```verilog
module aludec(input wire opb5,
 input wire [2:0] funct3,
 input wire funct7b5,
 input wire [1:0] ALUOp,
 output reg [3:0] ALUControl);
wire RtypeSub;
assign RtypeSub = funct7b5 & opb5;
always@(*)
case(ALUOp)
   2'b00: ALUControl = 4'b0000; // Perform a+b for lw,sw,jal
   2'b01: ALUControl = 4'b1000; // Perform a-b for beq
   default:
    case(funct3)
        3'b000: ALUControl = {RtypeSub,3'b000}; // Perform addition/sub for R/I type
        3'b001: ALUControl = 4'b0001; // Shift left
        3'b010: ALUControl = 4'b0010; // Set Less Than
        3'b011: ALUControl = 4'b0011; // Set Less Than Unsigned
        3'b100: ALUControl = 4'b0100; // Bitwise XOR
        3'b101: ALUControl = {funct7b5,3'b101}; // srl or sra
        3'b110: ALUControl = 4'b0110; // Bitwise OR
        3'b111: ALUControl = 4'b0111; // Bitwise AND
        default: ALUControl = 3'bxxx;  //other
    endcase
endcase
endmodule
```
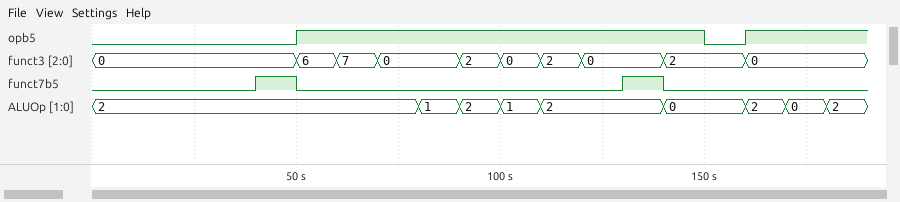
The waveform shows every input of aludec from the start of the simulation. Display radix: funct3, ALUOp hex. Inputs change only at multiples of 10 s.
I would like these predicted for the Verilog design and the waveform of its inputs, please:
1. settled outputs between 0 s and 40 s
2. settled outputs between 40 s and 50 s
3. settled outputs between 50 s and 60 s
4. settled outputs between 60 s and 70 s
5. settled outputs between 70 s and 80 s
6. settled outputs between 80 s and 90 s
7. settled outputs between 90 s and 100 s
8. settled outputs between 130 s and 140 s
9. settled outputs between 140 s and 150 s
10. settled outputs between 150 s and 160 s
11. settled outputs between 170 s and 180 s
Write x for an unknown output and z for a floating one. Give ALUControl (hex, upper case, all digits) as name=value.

ALUControl=0
ALUControl=0
ALUControl=6
ALUControl=7
ALUControl=0
ALUControl=8
ALUControl=2
ALUControl=8
ALUControl=0
ALUControl=0
ALUControl=0
